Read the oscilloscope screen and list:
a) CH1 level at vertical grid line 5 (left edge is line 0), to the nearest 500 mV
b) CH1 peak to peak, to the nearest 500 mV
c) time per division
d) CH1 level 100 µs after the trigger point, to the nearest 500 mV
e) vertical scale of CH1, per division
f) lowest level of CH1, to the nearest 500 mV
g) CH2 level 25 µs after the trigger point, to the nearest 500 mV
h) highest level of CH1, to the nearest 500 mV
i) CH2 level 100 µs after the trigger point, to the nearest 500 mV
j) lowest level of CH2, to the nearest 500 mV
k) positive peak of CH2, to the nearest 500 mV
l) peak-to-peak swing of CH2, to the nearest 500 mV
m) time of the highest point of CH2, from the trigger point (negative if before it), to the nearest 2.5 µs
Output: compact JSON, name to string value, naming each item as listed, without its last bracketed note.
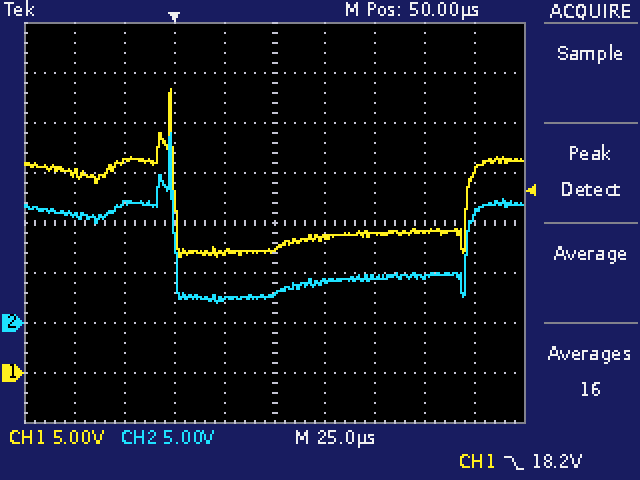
{"CH1 level at vertical grid line 5 (left edge is line 0), to the nearest 500 mV": "12.5 V", "CH1 peak to peak, to the nearest 500 mV": "17.0 V", "time per division": "25 µs", "CH1 level 100 µs after the trigger point, to the nearest 500 mV": "14.0 V", "vertical scale of CH1, per division": "5 V", "lowest level of CH1, to the nearest 500 mV": "11.5 V", "CH2 level 25 µs after the trigger point, to the nearest 500 mV": "2.5 V", "highest level of CH1, to the nearest 500 mV": "28.5 V", "CH2 level 100 µs after the trigger point, to the nearest 500 mV": "4.5 V", "lowest level of CH2, to the nearest 500 mV": "2.0 V", "positive peak of CH2, to the nearest 500 mV": "19.0 V", "peak-to-peak swing of CH2, to the nearest 500 mV": "17.0 V", "time of the highest point of CH2, from the trigger point (negative if before it), to the nearest 2.5 µs": "-2.5 µs"}
